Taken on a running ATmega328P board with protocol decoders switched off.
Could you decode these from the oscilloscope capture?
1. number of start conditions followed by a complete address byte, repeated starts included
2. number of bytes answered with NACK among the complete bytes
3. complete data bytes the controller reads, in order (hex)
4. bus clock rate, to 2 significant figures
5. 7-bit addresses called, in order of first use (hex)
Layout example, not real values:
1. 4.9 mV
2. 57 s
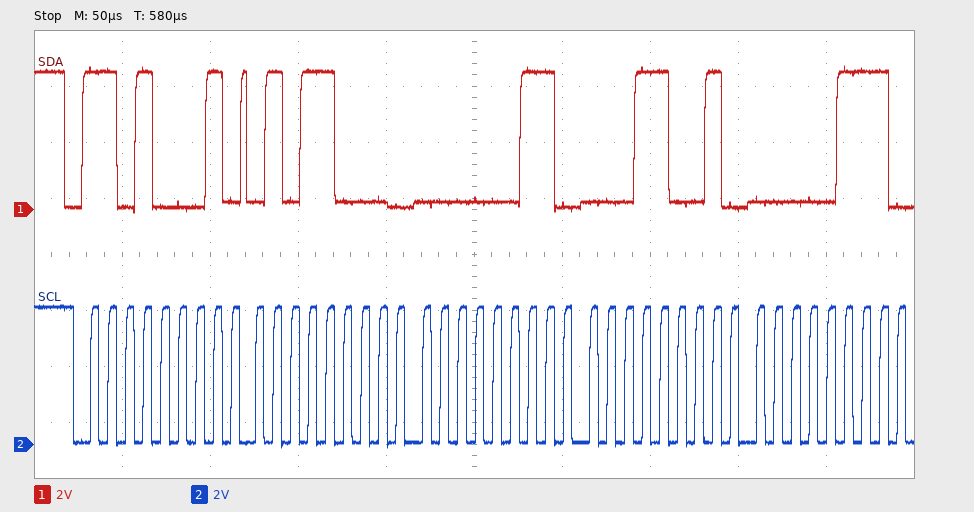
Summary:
1. 1
2. 0
3. 58 03 19 07
4. 100 kHz
5. 0x68
